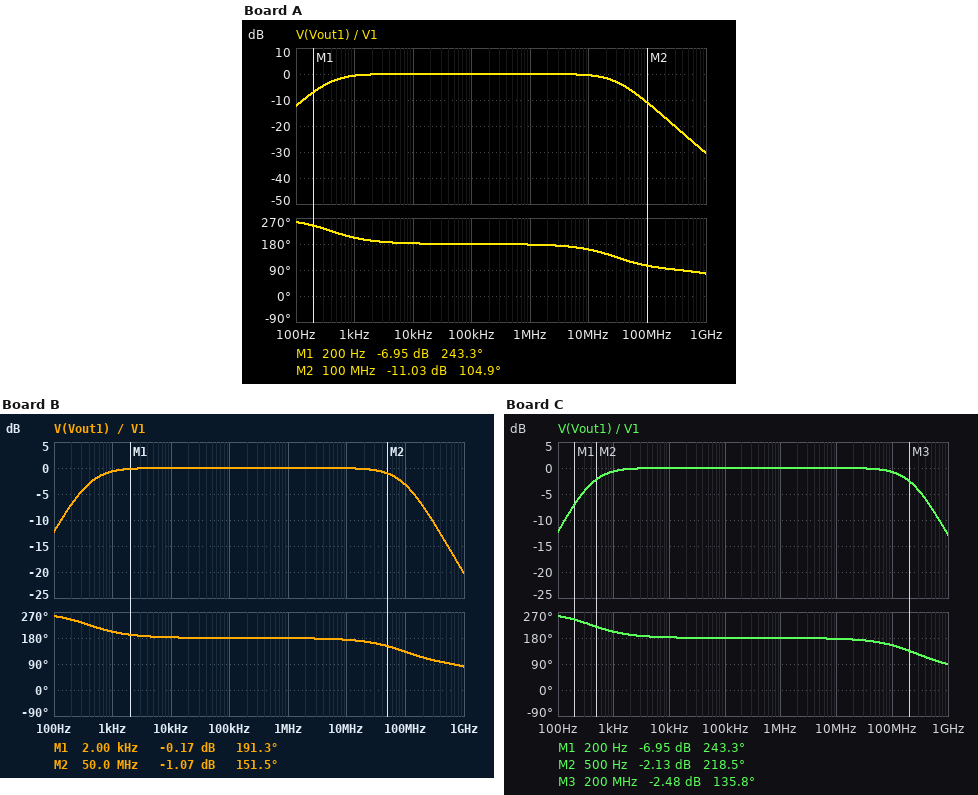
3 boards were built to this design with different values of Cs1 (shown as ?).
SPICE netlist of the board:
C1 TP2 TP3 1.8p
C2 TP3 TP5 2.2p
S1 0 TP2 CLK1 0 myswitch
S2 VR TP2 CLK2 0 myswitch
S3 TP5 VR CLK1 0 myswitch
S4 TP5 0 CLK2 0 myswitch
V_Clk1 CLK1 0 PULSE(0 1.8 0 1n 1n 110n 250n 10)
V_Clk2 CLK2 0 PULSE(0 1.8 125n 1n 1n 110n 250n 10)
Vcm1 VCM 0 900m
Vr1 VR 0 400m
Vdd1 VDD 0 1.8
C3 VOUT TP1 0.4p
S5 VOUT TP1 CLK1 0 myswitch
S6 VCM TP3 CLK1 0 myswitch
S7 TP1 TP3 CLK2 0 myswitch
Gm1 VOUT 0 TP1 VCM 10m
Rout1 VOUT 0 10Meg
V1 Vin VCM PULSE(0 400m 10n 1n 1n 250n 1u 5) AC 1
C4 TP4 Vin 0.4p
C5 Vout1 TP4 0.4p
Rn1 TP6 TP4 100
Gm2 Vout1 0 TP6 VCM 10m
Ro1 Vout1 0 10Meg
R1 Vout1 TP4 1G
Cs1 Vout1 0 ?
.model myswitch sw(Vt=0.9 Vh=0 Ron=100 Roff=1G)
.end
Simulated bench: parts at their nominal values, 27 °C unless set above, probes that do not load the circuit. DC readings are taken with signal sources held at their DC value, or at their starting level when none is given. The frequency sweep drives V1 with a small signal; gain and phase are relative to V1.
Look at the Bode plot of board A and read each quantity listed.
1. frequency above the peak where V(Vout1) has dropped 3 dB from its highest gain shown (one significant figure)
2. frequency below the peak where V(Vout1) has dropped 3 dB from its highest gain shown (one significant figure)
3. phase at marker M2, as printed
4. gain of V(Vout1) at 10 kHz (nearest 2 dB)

30 MHz
400 Hz
104.9 deg
0 dB
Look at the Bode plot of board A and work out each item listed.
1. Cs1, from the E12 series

27 pF
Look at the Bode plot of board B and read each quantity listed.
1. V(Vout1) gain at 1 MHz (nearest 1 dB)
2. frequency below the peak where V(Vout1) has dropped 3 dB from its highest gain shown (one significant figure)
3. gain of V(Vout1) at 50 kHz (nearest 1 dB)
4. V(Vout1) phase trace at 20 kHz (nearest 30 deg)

0 dB
400 Hz
0 dB
180 deg
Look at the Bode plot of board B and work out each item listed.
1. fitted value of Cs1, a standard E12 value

8.2 pF
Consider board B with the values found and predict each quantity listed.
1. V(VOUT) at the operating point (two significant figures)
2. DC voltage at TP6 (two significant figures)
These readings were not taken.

900 mV
900 mV
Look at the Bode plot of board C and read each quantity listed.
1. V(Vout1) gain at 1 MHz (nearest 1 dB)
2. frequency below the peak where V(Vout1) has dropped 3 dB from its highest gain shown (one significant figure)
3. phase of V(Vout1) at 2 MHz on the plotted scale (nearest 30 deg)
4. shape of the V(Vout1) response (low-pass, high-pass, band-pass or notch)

0 dB
400 Hz
180 deg
band-pass
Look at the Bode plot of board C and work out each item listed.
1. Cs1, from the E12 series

3.3 pF
